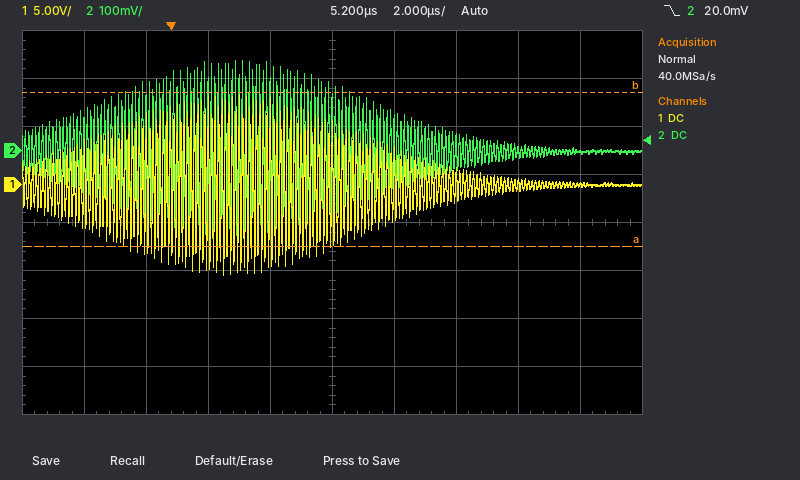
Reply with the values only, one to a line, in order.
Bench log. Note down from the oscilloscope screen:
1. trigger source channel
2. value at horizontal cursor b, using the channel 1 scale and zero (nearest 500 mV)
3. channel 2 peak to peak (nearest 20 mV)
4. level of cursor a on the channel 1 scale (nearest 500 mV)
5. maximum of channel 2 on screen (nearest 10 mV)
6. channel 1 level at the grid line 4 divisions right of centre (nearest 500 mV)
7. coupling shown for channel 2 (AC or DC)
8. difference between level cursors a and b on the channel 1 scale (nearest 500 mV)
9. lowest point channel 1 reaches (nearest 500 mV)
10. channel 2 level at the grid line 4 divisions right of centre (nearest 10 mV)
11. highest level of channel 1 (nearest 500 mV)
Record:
channel 2
9.5 V
380 mV
-6.5 V
190 mV
0.0 V
DC
16.0 V
-9.5 V
0 mV
9.5 V
